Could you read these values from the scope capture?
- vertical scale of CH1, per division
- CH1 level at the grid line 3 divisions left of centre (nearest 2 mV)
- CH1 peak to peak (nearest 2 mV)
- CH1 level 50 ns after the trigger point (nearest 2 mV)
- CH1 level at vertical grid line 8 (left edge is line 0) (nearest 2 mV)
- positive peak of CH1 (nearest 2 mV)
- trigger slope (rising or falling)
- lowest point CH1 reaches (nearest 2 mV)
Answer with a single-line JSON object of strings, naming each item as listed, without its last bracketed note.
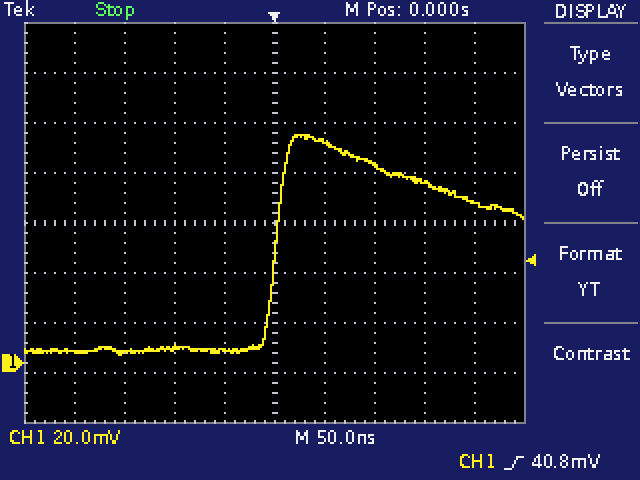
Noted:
{"vertical scale of CH1, per division": "20 mV", "CH1 level at the grid line 3 divisions left of centre": "4 mV", "CH1 peak to peak": "88 mV", "CH1 level 50 ns after the trigger point": "88 mV", "CH1 level at vertical grid line 8 (left edge is line 0)": "72 mV", "positive peak of CH1": "92 mV", "trigger slope": "rising", "lowest point CH1 reaches": "4 mV"}
